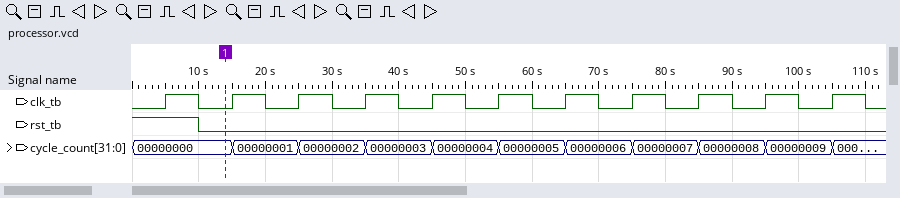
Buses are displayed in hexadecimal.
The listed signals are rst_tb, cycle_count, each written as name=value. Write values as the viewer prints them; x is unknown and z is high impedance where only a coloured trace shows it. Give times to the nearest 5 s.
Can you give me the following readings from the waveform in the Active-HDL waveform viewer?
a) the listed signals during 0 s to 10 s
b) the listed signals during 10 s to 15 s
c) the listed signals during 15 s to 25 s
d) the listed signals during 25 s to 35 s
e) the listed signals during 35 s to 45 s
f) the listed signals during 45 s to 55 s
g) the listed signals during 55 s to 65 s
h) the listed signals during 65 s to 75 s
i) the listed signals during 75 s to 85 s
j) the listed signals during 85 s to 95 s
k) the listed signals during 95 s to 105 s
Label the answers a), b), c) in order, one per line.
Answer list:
a) rst_tb=1, cycle_count=00000000
b) rst_tb=0, cycle_count=00000000
c) rst_tb=0, cycle_count=00000001
d) rst_tb=0, cycle_count=00000002
e) rst_tb=0, cycle_count=00000003
f) rst_tb=0, cycle_count=00000004
g) rst_tb=0, cycle_count=00000005
h) rst_tb=0, cycle_count=00000006
i) rst_tb=0, cycle_count=00000007
j) rst_tb=0, cycle_count=00000008
k) rst_tb=0, cycle_count=00000009
